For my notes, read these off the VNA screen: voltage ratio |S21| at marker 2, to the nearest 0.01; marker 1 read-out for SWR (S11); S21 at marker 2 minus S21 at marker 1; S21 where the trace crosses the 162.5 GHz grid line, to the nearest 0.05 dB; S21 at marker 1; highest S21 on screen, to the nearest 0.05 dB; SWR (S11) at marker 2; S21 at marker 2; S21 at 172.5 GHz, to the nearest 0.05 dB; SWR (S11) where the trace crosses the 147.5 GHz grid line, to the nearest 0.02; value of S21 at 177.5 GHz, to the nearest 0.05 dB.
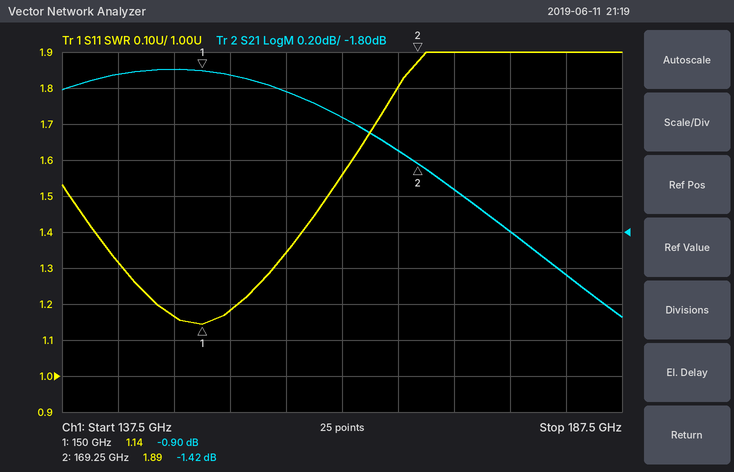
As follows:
0.85
1.14
-0.52 dB
-1.15 dB
-0.90 dB
-0.90 dB
1.89
-1.42 dB
-1.55 dB
1.16
-1.80 dB
